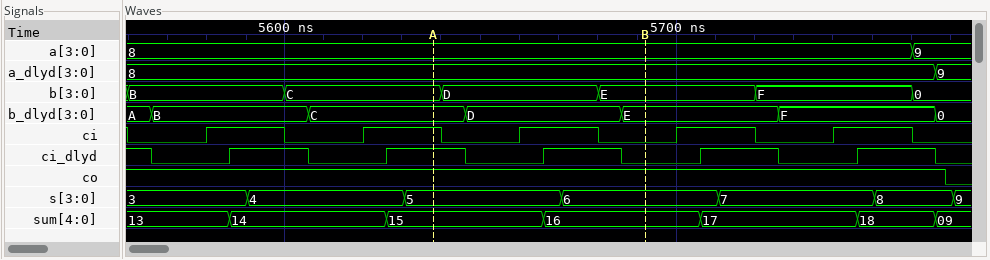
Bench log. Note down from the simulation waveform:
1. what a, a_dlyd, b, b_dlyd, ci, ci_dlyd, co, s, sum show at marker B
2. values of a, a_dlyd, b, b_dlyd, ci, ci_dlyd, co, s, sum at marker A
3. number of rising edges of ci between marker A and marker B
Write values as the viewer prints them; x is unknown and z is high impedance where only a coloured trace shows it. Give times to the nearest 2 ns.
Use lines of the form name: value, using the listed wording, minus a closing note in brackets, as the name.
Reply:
what a, a_dlyd, b, b_dlyd, ci, ci_dlyd, co, s, sum show at marker B: a=8, a_dlyd=8, b=E, b_dlyd=E, ci=0, ci_dlyd=0, co=1, s=6, sum=16
values of a, a_dlyd, b, b_dlyd, ci, ci_dlyd, co, s, sum at marker A: a=8, a_dlyd=8, b=C, b_dlyd=C, ci=1, ci_dlyd=1, co=1, s=5, sum=15
number of rising edges of ci between marker A and marker B: 1
